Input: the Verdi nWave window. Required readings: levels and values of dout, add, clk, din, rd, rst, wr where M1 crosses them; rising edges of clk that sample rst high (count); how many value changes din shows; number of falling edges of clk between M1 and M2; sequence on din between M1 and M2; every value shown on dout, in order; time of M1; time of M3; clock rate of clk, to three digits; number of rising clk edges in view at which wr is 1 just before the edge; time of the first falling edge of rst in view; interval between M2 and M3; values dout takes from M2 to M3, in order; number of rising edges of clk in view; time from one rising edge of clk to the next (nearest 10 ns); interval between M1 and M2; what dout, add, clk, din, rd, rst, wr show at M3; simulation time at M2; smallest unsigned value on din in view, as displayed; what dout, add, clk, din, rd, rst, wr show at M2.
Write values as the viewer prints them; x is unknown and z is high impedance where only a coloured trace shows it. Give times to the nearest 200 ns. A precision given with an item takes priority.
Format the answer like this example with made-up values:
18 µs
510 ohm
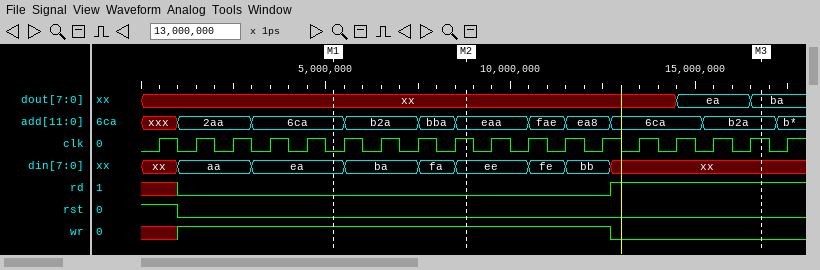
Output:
dout=xx, add=6ca, clk=0, din=ea, rd=0, rst=0, wr=1
1
8
3
ea, ba, fa, ee
xx, ea, ba
5200 ns
16800 ns
1.00 MHz
12
1000 ns
8000 ns
xx, ea, ba
18
1000 ns
3600 ns
dout=ba, add=b2a, clk=1, din=xx, rd=1, rst=0, wr=0
8800 ns
aa
dout=xx, add=eaa, clk=1, din=ee, rd=0, rst=0, wr=1
